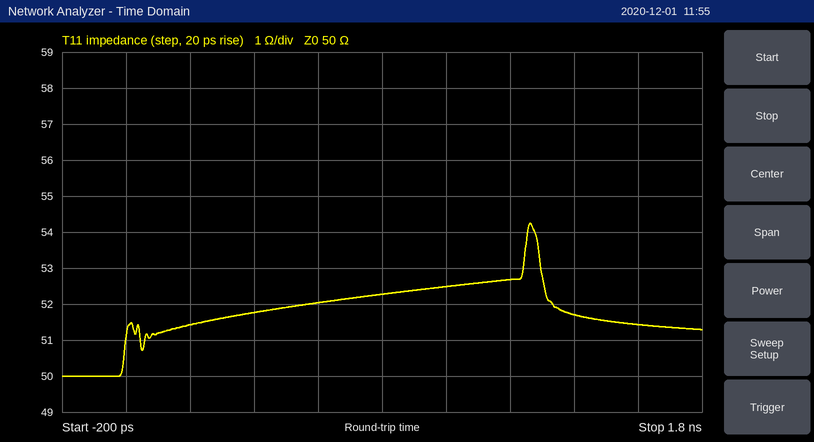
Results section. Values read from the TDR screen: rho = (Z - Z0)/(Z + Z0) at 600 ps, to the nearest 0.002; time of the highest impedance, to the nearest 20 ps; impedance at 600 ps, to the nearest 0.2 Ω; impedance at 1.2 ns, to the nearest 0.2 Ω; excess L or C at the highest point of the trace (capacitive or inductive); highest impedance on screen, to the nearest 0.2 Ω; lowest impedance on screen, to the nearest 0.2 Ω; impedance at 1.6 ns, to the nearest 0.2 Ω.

+0.020
1.26 ns
52.0 Ω
52.6 Ω
inductive
54.2 Ω
50.0 Ω
51.4 Ω
